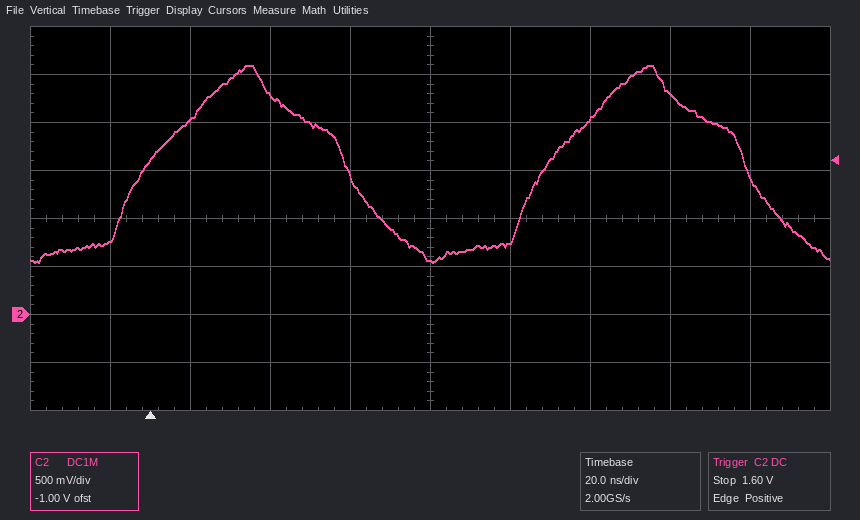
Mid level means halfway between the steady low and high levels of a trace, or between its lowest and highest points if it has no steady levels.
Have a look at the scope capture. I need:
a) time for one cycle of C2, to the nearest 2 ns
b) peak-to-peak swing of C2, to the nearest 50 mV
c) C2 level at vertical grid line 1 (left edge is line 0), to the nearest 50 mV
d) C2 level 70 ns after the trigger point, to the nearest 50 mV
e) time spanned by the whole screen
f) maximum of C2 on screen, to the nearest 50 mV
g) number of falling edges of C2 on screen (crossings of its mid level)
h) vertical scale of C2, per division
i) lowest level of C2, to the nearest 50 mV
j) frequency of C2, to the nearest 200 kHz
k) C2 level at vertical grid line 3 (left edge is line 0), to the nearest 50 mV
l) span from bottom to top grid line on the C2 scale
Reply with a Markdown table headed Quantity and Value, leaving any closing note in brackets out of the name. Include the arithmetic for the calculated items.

| Quantity | Value |
|---|---|
| time for one cycle of C2, to the nearest 2 ns | 100 ns |
| peak-to-peak swing of C2, to the nearest 50 mV | 2.60 V − (550 mV) = 2.05 V |
| C2 level at vertical grid line 1 (left edge is line 0), to the nearest 50 mV | 800 mV |
| C2 level 70 ns after the trigger point, to the nearest 50 mV | 550 mV |
| time spanned by the whole screen | 200 ns |
| maximum of C2 on screen, to the nearest 50 mV | 2.60 V |
| number of falling edges of C2 on screen | 2 |
| vertical scale of C2, per division | 500 mV |
| lowest level of C2, to the nearest 50 mV | 550 mV |
| frequency of C2, to the nearest 200 kHz | 1 / 100 ns ≈ 10.0 MHz |
| C2 level at vertical grid line 3 (left edge is line 0), to the nearest 50 mV | 2.30 V |
| span from bottom to top grid line on the C2 scale | 4 V |
